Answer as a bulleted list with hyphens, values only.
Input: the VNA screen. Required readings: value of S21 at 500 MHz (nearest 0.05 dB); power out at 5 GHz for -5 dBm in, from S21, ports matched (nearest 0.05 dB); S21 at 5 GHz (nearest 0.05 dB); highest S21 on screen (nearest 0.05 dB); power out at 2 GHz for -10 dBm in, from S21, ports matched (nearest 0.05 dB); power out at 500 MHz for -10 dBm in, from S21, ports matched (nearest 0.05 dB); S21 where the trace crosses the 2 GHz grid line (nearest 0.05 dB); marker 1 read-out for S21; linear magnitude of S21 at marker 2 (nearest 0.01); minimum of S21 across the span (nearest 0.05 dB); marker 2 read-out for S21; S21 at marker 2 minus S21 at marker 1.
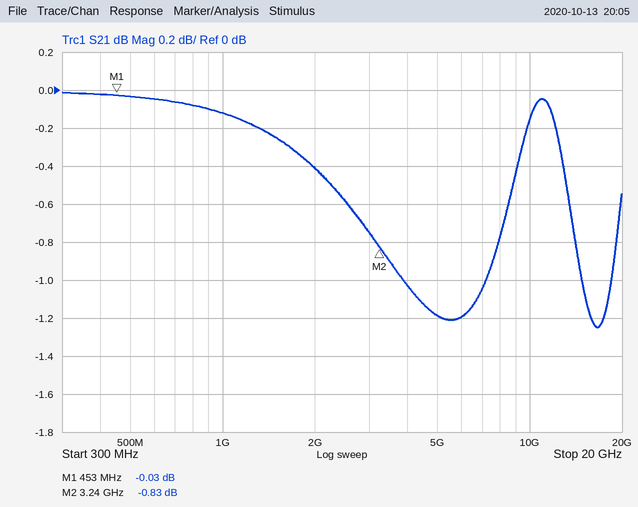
- -0.05 dB
- -6.20 dBm
- -1.20 dB
- 0.00 dB
- -10.40 dBm
- -10.05 dBm
- -0.40 dB
- -0.03 dB
- 0.91
- -1.25 dB
- -0.83 dB
- -0.80 dB
